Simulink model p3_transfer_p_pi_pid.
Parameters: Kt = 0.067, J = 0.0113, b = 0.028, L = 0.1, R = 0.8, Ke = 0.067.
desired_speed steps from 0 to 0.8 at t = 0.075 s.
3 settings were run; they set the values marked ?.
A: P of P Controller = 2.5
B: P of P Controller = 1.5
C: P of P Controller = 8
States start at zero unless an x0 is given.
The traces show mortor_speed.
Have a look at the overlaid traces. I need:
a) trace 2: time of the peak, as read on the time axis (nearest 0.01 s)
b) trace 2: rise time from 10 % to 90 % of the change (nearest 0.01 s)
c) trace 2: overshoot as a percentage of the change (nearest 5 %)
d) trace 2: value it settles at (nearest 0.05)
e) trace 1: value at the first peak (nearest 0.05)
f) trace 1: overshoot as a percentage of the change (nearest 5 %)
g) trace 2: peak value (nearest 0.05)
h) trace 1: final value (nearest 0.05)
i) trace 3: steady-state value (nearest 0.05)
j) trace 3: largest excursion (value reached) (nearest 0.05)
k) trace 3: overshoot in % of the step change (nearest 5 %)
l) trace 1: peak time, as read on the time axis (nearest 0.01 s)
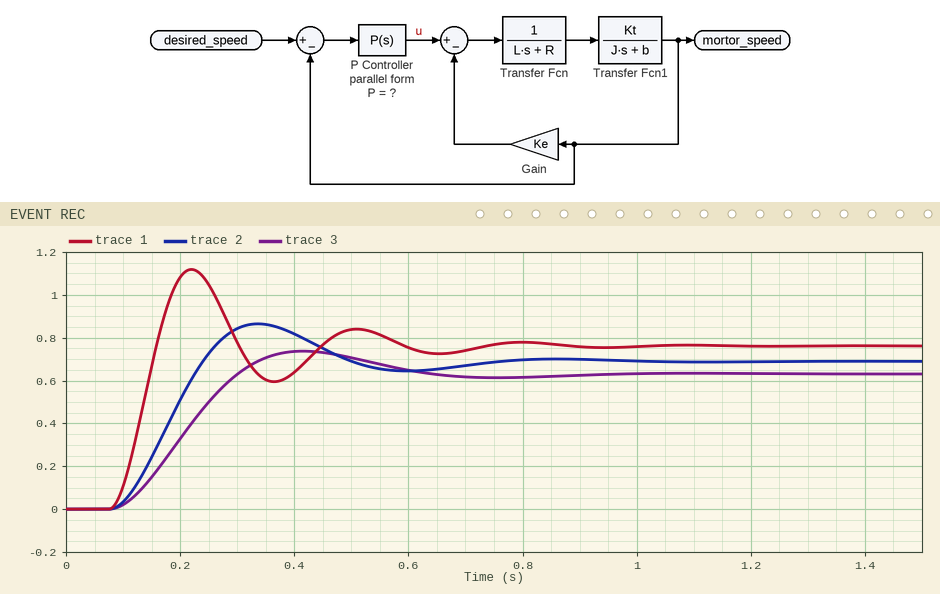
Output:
0.34 s
0.11 s
25 %
0.70
1.10
45 %
0.85
0.75
0.65
0.75
15 %
0.22 s
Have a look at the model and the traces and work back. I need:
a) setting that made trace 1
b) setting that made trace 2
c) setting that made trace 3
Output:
C
A
B
